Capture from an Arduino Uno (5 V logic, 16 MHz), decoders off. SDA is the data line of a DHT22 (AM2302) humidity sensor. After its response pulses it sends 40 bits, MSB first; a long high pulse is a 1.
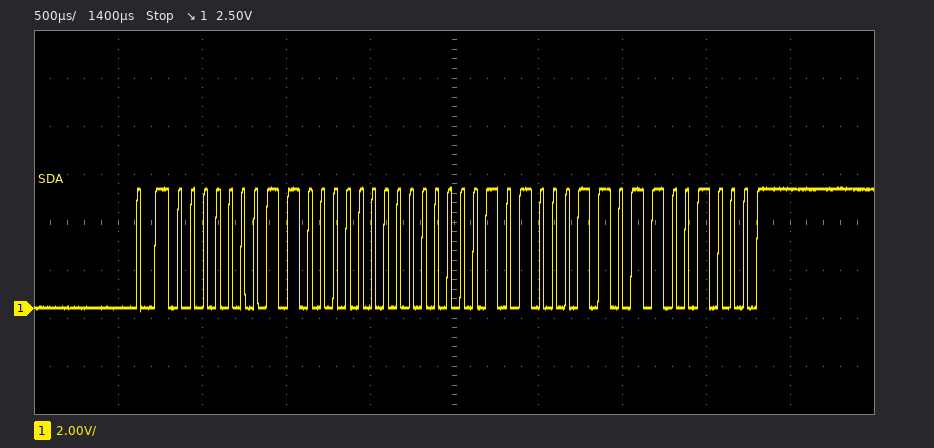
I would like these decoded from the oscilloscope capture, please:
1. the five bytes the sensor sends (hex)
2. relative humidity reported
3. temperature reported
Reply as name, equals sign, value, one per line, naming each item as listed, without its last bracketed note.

the five bytes the sensor sends = 01 80 01 46 C8
relative humidity reported = 38.4 %
temperature reported = 32.6 °C
